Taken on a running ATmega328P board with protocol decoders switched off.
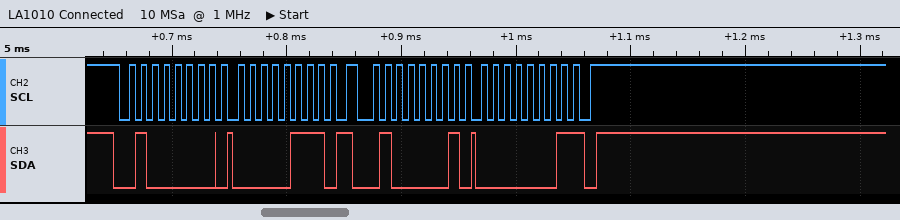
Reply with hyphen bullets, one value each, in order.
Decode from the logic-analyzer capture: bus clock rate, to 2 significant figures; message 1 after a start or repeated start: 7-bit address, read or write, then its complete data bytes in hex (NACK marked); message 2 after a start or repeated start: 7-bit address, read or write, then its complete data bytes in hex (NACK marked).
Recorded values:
- 100 kHz
- 0x20 write: 07
- 0x20 read: 01 NACK
